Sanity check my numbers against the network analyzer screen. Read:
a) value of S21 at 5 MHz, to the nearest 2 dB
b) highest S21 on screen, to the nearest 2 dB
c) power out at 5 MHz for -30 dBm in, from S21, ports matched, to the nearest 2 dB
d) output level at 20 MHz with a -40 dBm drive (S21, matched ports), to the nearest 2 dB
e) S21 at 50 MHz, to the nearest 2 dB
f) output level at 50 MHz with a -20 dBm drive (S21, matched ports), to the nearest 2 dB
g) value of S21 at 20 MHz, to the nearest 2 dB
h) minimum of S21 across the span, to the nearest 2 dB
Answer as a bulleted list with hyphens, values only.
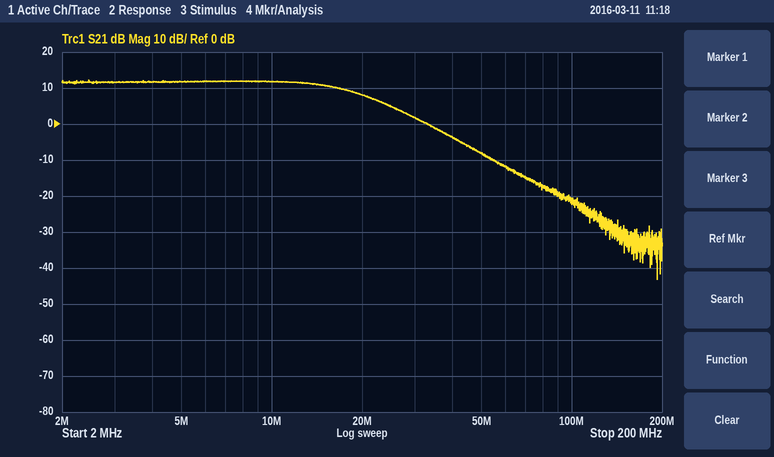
- 12 dB
- 12 dB
- -18 dBm
- -32 dBm
- -8 dB
- -28 dBm
- 8 dB
- -44 dB
